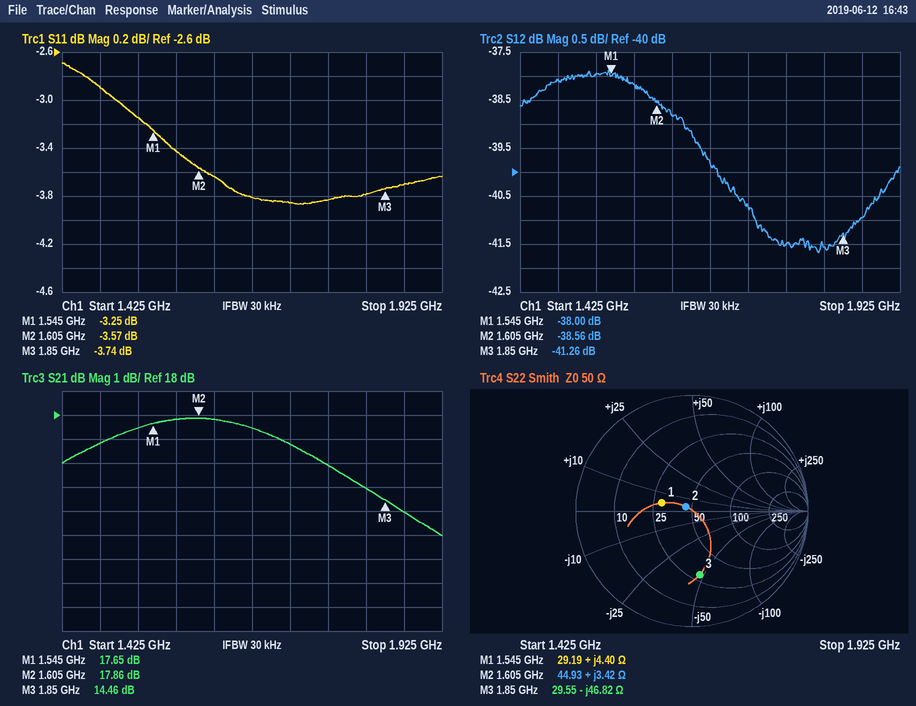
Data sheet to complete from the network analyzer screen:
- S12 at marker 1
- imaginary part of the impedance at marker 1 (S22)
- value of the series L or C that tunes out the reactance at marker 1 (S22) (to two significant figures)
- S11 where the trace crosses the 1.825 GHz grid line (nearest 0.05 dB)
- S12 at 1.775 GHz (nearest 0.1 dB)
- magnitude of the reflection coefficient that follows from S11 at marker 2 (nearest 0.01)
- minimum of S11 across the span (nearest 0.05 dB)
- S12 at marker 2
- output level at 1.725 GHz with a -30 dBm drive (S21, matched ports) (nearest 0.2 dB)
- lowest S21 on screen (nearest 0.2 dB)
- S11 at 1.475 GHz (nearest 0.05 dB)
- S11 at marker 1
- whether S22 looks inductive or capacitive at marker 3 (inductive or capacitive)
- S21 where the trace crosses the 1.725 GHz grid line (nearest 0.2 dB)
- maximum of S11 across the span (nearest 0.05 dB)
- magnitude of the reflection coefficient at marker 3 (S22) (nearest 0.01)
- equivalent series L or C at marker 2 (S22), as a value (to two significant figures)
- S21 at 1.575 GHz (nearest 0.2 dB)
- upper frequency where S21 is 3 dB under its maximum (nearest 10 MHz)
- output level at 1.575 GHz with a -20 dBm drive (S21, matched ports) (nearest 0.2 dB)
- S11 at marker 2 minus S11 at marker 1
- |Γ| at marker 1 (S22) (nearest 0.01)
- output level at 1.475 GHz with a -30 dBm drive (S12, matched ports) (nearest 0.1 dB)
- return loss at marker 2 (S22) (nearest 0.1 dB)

-38.00 dB
+4.40 Ω
23 pF
-3.80 dB
-41.5 dB
0.66
-3.85 dB
-38.56 dB
-13.2 dBm
13.0 dB
-2.90 dB
-3.25 dB
capacitive
16.8 dB
-2.70 dB
0.55
340 pH
17.8 dB
1.83 GHz
-2.2 dBm
-0.32 dB
0.27
-68.1 dBm
23.8 dB
